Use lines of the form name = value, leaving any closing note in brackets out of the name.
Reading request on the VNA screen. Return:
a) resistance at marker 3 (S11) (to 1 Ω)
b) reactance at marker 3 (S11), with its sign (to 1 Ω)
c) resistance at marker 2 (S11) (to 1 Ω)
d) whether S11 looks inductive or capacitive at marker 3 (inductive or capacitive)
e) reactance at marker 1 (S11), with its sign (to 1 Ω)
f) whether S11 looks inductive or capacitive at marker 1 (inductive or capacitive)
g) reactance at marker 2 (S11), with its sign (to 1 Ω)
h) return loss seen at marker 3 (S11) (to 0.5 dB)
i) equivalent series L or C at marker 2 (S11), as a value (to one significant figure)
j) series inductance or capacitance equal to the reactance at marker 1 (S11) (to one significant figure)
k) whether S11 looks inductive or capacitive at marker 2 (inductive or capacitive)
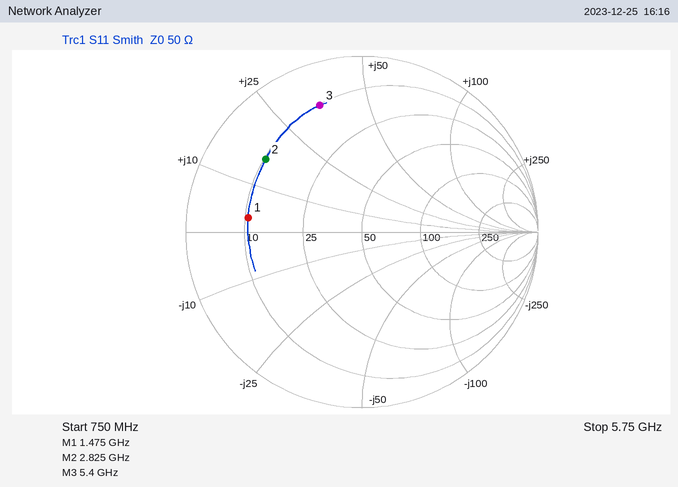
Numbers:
resistance at marker 3 (S11) = 10 Ω
reactance at marker 3 (S11), with its sign = +35 Ω
resistance at marker 2 (S11) = 10 Ω
whether S11 looks inductive or capacitive at marker 3 = inductive
reactance at marker 1 (S11), with its sign = +3 Ω
whether S11 looks inductive or capacitive at marker 1 = inductive
reactance at marker 2 (S11), with its sign = +16 Ω
return loss seen at marker 3 (S11) = 2.5 dB
equivalent series L or C at marker 2 (S11), as a value = 900 pH
series inductance or capacitance equal to the reactance at marker 1 (S11) = 300 pH
whether S11 looks inductive or capacitive at marker 2 = inductive
